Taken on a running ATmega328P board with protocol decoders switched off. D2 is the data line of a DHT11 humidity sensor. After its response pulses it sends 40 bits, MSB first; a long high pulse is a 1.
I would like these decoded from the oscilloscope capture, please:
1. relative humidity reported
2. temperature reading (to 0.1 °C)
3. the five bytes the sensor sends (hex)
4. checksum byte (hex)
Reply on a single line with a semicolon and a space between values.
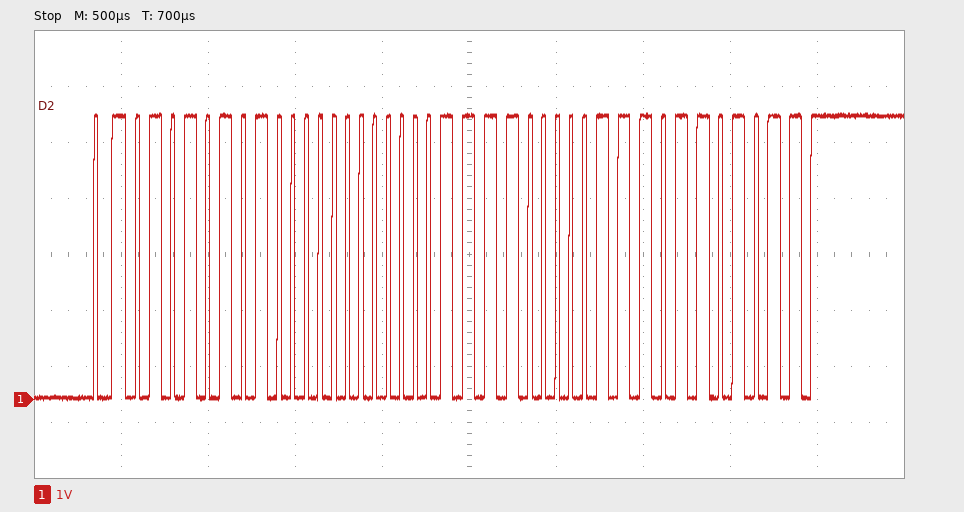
85 %; 15.7 °C; 55 00 0F 07 6B; 0x6B
